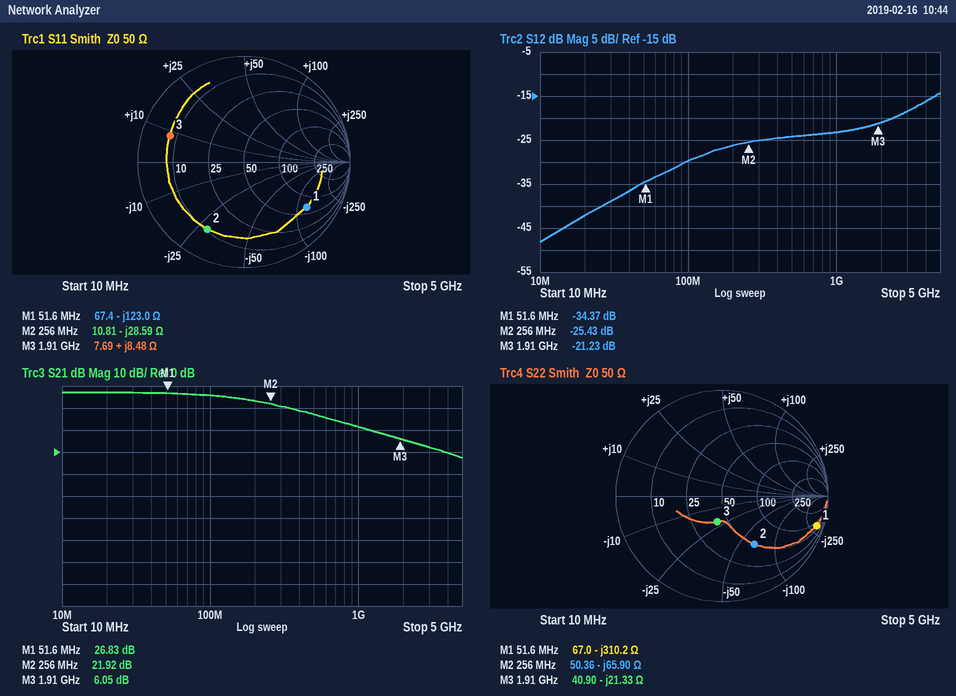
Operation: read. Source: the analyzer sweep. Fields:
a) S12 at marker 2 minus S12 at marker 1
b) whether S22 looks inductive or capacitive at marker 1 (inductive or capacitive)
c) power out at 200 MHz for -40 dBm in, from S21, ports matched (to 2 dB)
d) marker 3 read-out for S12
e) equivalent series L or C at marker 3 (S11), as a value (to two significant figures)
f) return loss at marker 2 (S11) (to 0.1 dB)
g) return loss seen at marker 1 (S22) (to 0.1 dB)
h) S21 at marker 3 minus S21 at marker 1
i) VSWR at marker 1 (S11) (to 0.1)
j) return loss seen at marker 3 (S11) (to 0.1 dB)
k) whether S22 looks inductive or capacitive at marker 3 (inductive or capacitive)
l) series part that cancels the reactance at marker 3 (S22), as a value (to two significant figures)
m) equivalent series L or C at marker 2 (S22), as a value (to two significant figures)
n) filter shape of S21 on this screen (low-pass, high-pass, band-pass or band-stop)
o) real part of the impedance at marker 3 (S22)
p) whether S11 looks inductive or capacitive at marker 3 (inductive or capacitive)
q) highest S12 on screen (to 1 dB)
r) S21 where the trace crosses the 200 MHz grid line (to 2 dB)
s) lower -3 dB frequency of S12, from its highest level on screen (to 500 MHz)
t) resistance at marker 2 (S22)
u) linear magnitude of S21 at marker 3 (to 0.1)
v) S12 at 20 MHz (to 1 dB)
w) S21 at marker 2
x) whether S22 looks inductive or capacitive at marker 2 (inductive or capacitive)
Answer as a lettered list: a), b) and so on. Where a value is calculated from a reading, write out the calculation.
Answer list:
a) -25.43 − (-34.37) = 8.94 dB
b) capacitive
c) -40 dBm + (24 dB) = -16 dBm
d) -21.23 dB
e) L = 8.48 Ω/(2π × 1.91 GHz) ≈ 707 pH, so 710 pH to two significant figures
f) 2.8 dB
g) 0.6 dB
h) 6.05 − (26.83) = -20.78 dB
i) 6.4
j) 2.6 dB
k) capacitive
l) L = 21.33 Ω/(2π × 1.91 GHz) ≈ 1.8 nH
m) C = 1/(2π × 256 MHz × 65.9 Ω) ≈ 9.4 pF
n) low-pass
o) 40.90 Ω
p) inductive
q) -14 dB
r) 24 dB
s) 3.5 GHz
t) 50.36 Ω
u) 10^(6.05/20) ≈ 2.0
v) -42 dB
w) 21.92 dB
x) capacitive
